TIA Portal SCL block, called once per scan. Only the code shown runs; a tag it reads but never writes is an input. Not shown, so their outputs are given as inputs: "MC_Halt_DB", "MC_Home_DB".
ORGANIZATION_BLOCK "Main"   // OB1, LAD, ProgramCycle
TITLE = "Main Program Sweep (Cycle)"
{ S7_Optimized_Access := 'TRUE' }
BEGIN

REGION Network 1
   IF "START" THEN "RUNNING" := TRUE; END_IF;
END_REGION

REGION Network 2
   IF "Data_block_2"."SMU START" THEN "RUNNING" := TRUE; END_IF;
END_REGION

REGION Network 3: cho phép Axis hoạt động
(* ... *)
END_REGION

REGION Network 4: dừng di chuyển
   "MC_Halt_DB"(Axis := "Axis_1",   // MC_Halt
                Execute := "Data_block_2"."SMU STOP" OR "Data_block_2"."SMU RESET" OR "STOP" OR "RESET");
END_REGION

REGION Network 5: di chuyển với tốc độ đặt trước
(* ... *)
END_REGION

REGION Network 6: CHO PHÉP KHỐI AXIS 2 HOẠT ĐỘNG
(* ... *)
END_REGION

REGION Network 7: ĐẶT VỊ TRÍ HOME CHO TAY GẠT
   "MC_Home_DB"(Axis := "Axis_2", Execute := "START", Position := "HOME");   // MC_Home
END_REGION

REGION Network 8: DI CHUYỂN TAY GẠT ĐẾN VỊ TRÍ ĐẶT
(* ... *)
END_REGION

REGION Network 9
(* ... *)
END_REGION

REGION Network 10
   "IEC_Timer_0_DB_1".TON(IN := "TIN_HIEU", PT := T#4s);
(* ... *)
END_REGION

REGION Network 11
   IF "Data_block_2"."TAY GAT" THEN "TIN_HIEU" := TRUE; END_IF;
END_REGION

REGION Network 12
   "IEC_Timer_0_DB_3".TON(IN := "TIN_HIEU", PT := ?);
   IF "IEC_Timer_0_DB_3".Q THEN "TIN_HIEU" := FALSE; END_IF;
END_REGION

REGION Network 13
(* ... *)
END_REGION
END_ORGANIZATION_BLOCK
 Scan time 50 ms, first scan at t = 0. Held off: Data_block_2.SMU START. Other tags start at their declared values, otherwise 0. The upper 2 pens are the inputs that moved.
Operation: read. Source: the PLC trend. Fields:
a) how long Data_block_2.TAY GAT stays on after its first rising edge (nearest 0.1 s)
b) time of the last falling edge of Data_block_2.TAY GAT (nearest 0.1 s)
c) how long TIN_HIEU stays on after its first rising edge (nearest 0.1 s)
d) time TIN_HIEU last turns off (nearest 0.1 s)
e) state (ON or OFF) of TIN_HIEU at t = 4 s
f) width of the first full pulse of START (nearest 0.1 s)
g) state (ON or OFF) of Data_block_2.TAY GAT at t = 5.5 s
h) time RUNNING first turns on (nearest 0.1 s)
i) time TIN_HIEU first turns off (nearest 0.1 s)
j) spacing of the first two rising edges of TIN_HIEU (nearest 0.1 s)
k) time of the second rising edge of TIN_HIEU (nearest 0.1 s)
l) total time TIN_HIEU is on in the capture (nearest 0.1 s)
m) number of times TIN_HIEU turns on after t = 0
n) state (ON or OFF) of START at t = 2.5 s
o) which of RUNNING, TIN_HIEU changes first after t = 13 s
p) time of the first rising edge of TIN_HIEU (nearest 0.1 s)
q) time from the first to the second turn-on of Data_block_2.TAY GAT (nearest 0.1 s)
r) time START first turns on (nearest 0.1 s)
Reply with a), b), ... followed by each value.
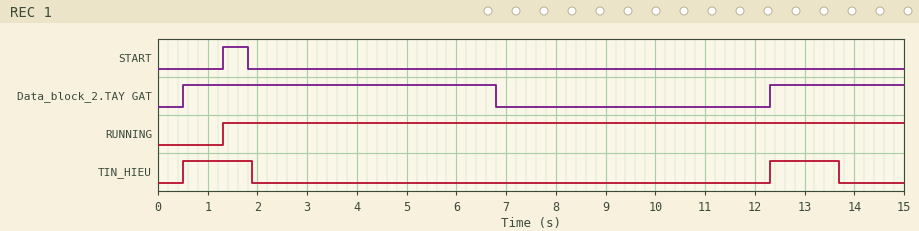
a) 6.3 s
b) 6.8 s
c) 1.4 s
d) 13.7 s
e) OFF
f) 0.5 s
g) ON
h) 1.3 s
i) 1.9 s
j) 11.8 s
k) 12.3 s
l) 2.8 s
m) 2
n) OFF
o) TIN_HIEU
p) 0.5 s
q) 11.8 s
r) 1.3 s
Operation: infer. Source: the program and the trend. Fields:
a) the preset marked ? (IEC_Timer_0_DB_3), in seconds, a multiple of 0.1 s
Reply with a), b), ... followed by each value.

a) 1.4 s
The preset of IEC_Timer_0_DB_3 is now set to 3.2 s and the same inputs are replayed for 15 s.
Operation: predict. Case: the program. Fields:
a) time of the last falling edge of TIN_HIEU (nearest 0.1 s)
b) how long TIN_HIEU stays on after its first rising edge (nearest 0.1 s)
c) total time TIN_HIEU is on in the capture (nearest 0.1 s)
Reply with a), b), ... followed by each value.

a) 3.7 s
b) 3.2 s
c) 5.9 s
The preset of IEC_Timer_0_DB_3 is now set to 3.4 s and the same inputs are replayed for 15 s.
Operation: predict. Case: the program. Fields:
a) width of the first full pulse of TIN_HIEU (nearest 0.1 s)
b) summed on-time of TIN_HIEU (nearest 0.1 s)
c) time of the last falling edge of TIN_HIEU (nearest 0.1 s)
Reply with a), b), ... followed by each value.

a) 3.4 s
b) 6.1 s
c) 3.9 s
